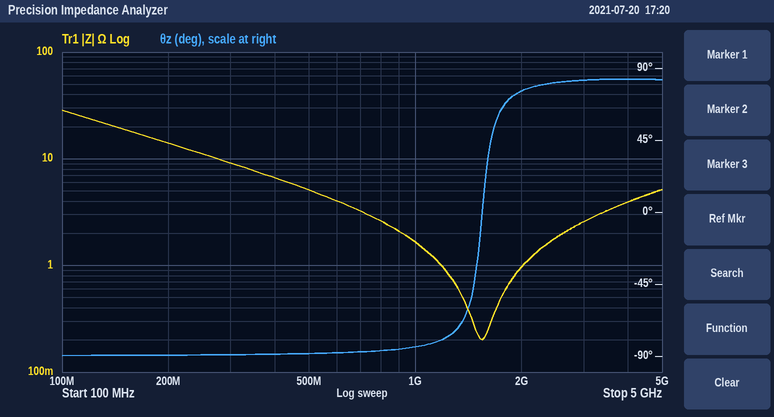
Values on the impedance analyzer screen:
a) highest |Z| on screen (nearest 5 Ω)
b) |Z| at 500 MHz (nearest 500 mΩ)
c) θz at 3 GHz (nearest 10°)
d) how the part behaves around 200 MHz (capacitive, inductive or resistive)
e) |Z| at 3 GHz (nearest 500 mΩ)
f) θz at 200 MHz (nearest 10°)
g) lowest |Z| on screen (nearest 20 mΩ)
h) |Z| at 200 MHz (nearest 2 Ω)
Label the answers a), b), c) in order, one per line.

a) 30 Ω
b) 5.0 Ω
c) 80°
d) capacitive
e) 2.5 Ω
f) -90°
g) 200 mΩ
h) 14 Ω
